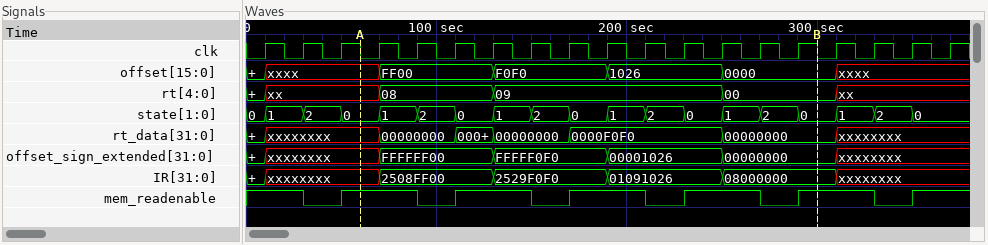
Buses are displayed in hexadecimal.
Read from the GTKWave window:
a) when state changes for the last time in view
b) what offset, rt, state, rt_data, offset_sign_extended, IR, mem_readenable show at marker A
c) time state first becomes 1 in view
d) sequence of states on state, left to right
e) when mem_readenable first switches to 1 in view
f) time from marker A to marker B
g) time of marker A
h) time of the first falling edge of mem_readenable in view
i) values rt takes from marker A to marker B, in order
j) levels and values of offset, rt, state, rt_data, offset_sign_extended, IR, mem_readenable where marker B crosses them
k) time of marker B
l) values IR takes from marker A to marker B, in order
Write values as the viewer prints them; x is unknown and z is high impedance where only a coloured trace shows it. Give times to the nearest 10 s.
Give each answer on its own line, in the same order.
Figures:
350 s
offset=xxxx, rt=xx, state=0, rt_data=xxxxxxxx, offset_sign_extended=xxxxxxxx, IR=xxxxxxxx, mem_readenable=1
10 s
0, 1, 2, 0, 1, 2, 0, 1, 2, 0, 1, 2, 0, 1, 2, 0, 1, 2, 0
50 s
240 s
60 s
30 s
xx, 08, 09, 00
offset=0000, rt=00, state=0, rt_data=00000000, offset_sign_extended=00000000, IR=08000000, mem_readenable=1
300 s
xxxxxxxx, 2508FF00, 2529F0F0, 01091026, 08000000
